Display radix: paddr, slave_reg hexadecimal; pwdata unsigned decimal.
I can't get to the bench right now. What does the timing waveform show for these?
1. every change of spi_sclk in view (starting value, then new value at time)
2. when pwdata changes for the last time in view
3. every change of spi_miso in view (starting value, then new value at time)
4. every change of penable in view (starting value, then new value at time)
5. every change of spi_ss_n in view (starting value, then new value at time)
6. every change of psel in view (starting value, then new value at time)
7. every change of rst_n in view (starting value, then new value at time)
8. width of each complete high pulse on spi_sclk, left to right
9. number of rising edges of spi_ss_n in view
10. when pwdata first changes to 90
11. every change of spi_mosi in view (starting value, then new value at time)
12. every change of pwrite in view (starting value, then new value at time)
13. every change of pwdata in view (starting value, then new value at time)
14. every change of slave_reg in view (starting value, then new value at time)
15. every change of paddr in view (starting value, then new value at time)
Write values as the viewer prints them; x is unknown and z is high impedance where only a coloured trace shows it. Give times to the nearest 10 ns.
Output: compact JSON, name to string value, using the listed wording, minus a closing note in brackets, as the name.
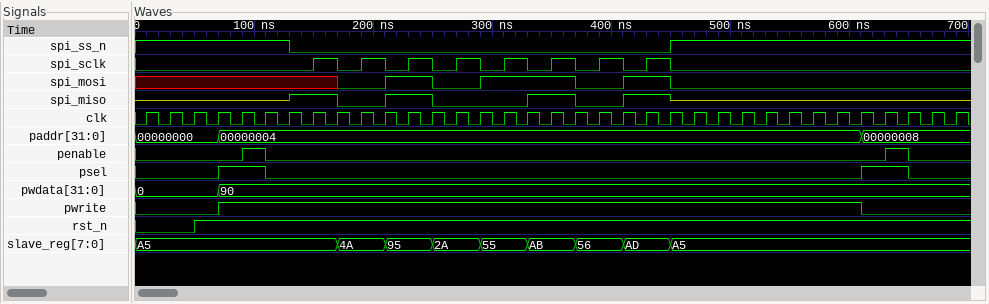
{"every change of spi_sclk in view": "0, 1 at 150 ns, 0 at 170 ns, 1 at 190 ns, 0 at 210 ns, 1 at 230 ns, 0 at 250 ns, 1 at 270 ns, 0 at 290 ns, 1 at 310 ns, 0 at 330 ns, 1 at 350 ns, 0 at 370 ns, 1 at 390 ns, 0 at 410 ns, 1 at 430 ns, 0 at 450 ns", "when pwdata changes for the last time in view": "70 ns", "every change of spi_miso in view": "z, 1 at 130 ns, 0 at 170 ns, 1 at 210 ns, 0 at 250 ns, 1 at 330 ns, 0 at 370 ns, 1 at 410 ns, z at 450 ns", "every change of penable in view": "0, 1 at 90 ns, 0 at 110 ns, 1 at 630 ns, 0 at 650 ns", "every change of spi_ss_n in view": "1, 0 at 130 ns, 1 at 450 ns", "every change of psel in view": "0, 1 at 70 ns, 0 at 110 ns, 1 at 610 ns, 0 at 650 ns", "every change of rst_n in view": "0, 1 at 50 ns", "width of each complete high pulse on spi_sclk, left to right": "20 ns, 20 ns, 20 ns, 20 ns, 20 ns, 20 ns, 20 ns, 20 ns", "number of rising edges of spi_ss_n in view": "1", "when pwdata first changes to 90": "70 ns", "every change of spi_mosi in view": "x, 0 at 170 ns, 1 at 210 ns, 0 at 250 ns, 1 at 290 ns, 0 at 370 ns, 1 at 410 ns, 0 at 450 ns", "every change of pwrite in view": "0, 1 at 70 ns, 0 at 610 ns", "every change of pwdata in view": "0, 90 at 70 ns", "every change of slave_reg in view": "A5, 4A at 170 ns, 95 at 210 ns, 2A at 250 ns, 55 at 290 ns, AB at 330 ns, 56 at 370 ns, AD at 410 ns, A5 at 450 ns", "every change of paddr in view": "00000000, 00000004 at 70 ns, 00000008 at 610 ns"}
